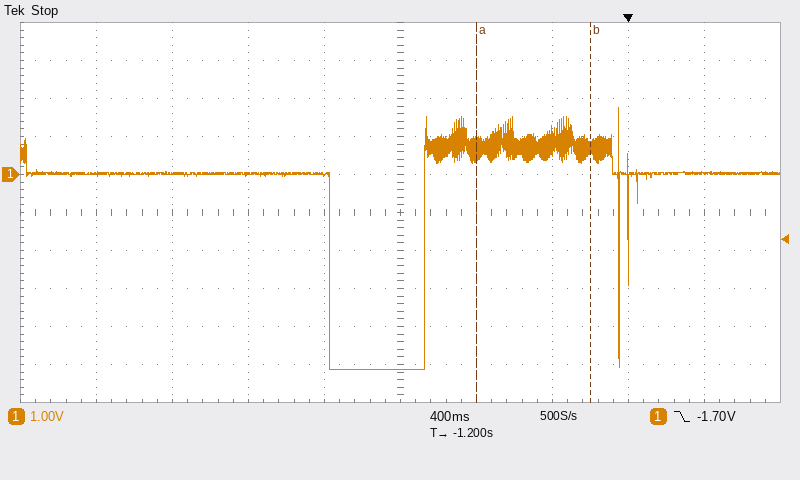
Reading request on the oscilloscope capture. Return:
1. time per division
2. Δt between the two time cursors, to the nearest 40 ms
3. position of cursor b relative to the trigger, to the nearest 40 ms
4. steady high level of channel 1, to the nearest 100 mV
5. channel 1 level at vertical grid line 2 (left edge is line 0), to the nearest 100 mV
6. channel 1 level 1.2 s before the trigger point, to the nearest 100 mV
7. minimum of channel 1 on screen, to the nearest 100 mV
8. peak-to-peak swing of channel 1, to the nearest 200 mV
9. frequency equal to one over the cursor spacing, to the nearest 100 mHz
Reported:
400 ms
600 ms
-200 ms
0.0 V
0.0 V
-5.1 V
-5.1 V
6.8 V
1.7 Hz
